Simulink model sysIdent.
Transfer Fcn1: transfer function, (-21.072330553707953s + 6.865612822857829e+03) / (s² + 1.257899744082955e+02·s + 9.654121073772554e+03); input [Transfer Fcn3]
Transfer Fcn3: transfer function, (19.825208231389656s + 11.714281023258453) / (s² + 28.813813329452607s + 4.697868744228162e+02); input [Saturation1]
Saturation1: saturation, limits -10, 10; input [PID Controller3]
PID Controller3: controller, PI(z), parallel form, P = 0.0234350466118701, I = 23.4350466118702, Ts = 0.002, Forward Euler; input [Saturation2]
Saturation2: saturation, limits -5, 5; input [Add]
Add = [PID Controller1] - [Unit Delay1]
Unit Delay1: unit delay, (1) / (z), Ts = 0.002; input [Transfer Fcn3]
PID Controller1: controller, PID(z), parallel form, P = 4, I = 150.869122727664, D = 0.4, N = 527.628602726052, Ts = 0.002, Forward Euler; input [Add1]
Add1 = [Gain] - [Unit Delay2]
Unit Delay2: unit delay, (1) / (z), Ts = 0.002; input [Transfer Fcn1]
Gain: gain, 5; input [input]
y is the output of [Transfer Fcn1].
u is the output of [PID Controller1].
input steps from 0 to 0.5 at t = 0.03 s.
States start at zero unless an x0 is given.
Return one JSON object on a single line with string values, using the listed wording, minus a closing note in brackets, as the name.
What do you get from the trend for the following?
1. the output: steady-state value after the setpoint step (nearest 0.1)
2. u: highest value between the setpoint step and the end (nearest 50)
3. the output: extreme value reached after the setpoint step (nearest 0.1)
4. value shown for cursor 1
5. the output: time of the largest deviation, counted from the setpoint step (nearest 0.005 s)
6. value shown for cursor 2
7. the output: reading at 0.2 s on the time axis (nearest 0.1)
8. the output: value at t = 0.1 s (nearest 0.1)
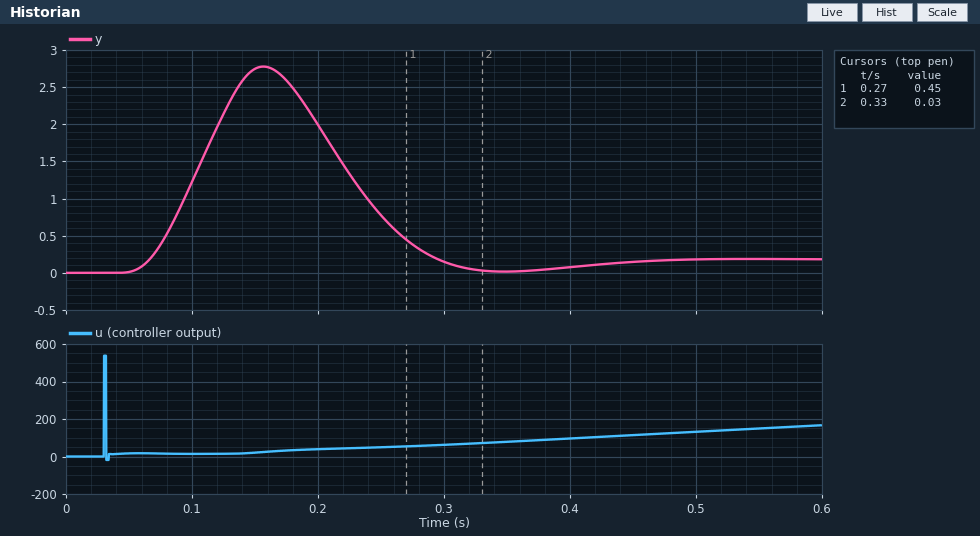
{"the output: steady-state value after the setpoint step": "0.2", "u: highest value between the setpoint step and the end": "550", "the output: extreme value reached after the setpoint step": "2.8", "value shown for cursor 1": "0.45", "the output: time of the largest deviation, counted from the setpoint step": "0.125 s", "value shown for cursor 2": "0.03", "the output: reading at 0.2 s on the time axis": "2.0", "the output: value at t = 0.1 s": "1.2"}
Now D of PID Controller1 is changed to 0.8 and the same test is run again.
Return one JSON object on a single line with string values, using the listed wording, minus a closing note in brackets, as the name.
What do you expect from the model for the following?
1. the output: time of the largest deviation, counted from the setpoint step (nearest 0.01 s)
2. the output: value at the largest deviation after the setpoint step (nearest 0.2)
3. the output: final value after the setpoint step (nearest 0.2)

{"the output: time of the largest deviation, counted from the setpoint step": "0.15 s", "the output: value at the largest deviation after the setpoint step": "2.4", "the output: final value after the setpoint step": "0.2"}
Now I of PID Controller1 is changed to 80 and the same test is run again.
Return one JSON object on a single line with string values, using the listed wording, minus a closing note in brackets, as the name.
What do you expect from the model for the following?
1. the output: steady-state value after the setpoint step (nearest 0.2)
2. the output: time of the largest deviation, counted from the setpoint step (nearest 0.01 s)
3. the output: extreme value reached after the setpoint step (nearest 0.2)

{"the output: steady-state value after the setpoint step": "0.2", "the output: time of the largest deviation, counted from the setpoint step": "0.14 s", "the output: extreme value reached after the setpoint step": "2.4"}
